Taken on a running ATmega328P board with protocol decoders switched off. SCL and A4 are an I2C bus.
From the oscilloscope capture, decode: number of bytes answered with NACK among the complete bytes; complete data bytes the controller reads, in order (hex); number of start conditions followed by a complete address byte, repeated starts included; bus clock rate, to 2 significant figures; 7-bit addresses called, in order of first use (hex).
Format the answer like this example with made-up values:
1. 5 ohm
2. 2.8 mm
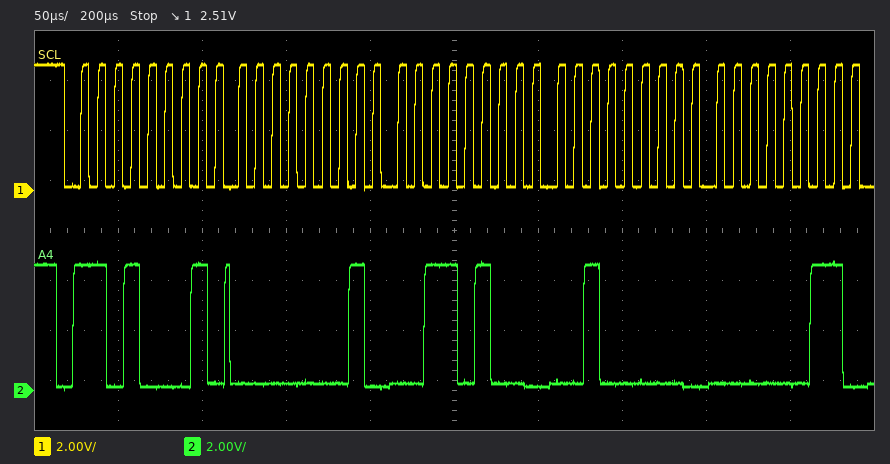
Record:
1. 0
2. 01 34 20 03
3. 1
4. 100 kHz
5. 0x68
